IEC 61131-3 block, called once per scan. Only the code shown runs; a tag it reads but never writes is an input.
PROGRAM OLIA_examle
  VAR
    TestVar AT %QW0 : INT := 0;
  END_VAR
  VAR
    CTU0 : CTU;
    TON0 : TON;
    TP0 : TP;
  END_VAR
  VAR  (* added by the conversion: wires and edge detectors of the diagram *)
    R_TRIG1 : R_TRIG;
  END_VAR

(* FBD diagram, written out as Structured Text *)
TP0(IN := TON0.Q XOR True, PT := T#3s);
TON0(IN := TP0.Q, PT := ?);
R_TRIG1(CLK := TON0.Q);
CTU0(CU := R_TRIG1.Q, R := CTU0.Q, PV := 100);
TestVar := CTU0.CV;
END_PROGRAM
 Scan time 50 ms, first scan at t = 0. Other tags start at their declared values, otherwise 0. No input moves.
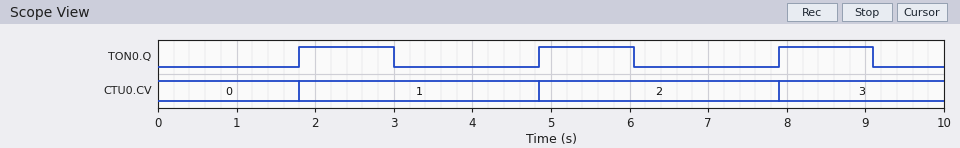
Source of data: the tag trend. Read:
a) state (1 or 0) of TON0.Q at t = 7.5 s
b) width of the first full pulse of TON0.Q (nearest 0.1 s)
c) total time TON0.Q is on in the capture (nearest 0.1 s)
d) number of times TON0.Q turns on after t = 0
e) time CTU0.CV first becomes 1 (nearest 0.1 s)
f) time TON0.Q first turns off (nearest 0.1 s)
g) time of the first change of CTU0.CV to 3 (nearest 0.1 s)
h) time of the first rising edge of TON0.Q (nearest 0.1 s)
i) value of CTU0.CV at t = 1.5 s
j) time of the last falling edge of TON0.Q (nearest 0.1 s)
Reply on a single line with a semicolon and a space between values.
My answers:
0; 1.2 s; 3.6 s; 3; 1.8 s; 3.0 s; 7.9 s; 1.8 s; 0; 9.1 s
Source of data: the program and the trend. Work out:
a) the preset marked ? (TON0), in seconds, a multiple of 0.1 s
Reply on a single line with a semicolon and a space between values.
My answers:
1.8 s
